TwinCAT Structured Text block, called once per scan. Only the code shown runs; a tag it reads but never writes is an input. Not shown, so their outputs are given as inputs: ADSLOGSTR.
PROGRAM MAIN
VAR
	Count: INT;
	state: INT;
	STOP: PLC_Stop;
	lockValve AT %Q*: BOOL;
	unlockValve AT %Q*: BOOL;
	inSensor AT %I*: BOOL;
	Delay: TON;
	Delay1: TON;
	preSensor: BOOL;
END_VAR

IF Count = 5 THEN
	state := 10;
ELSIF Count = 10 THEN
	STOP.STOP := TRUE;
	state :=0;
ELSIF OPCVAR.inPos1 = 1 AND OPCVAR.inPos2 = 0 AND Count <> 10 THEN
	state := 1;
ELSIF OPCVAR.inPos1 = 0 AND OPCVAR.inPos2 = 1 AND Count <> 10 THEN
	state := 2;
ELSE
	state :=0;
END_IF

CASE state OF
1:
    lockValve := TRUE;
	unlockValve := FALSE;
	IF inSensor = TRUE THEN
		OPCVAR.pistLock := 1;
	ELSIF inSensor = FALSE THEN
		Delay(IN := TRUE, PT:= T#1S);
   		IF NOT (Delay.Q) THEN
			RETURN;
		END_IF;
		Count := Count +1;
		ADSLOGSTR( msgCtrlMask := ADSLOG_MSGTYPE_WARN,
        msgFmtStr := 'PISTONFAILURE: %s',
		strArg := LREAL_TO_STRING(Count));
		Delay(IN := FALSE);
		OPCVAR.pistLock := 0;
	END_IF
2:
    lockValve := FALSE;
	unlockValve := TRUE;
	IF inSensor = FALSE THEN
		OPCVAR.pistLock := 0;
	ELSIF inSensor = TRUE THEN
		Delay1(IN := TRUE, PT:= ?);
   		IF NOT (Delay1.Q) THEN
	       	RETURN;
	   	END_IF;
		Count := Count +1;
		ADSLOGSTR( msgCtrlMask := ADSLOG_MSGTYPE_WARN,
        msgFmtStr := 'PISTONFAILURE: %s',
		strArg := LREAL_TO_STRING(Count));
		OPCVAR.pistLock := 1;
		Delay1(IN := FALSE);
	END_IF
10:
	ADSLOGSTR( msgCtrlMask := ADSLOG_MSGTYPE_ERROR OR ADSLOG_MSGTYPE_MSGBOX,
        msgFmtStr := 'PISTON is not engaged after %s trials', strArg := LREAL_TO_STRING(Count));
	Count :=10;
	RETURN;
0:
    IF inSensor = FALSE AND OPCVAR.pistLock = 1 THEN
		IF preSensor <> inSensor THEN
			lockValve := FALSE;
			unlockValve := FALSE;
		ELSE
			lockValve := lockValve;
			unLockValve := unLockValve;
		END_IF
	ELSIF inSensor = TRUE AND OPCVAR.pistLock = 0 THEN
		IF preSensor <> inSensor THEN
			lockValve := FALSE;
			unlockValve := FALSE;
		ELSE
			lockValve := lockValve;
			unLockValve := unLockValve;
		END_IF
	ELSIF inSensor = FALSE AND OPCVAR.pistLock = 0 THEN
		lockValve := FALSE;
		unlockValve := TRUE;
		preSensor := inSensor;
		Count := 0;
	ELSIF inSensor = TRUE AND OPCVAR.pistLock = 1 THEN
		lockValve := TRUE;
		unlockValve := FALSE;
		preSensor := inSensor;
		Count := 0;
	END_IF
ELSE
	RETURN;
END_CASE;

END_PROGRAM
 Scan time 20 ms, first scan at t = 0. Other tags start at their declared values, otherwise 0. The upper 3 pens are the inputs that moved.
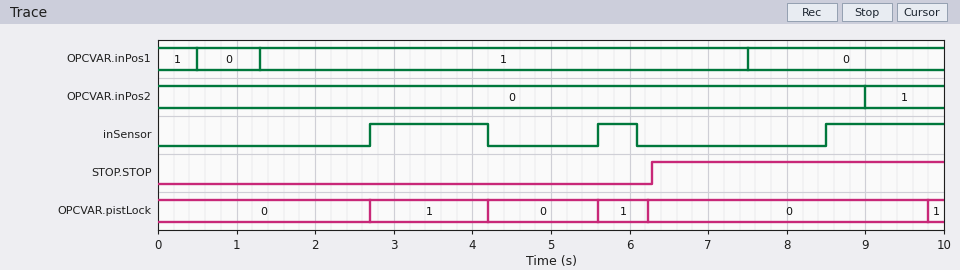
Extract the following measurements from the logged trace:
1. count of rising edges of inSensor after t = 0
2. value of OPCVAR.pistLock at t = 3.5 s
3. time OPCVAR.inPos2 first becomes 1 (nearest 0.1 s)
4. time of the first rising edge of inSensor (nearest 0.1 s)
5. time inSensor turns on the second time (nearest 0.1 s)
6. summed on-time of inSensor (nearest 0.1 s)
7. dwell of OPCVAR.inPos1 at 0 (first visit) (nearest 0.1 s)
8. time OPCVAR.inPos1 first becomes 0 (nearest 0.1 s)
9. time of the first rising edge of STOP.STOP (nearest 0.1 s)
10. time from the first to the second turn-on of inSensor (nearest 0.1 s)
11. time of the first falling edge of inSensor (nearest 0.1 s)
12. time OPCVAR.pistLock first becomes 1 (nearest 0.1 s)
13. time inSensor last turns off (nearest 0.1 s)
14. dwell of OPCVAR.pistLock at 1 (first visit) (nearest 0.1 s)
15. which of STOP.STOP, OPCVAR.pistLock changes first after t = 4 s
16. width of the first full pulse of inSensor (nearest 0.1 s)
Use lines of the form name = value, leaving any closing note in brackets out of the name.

count of rising edges of inSensor after t = 0 = 3
value of OPCVAR.pistLock at t = 3.5 s = 1
time OPCVAR.inPos2 first becomes 1 = 9.0 s
time of the first rising edge of inSensor = 2.7 s
time inSensor turns on the second time = 5.6 s
summed on-time of inSensor = 3.5 s
dwell of OPCVAR.inPos1 at 0 (first visit) = 0.8 s
time OPCVAR.inPos1 first becomes 0 = 0.5 s
time of the first rising edge of STOP.STOP = 6.3 s
time from the first to the second turn-on of inSensor = 2.9 s
time of the first falling edge of inSensor = 4.2 s
time OPCVAR.pistLock first becomes 1 = 2.7 s
time inSensor last turns off = 6.1 s
dwell of OPCVAR.pistLock at 1 (first visit) = 1.5 s
which of STOP.STOP, OPCVAR.pistLock changes first after t = 4 s = OPCVAR.pistLock
width of the first full pulse of inSensor = 1.5 s
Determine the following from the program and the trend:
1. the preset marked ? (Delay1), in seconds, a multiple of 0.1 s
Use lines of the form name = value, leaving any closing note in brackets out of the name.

the preset marked ? (Delay1), in seconds, a multiple of 0.1 s = 0.8 s
